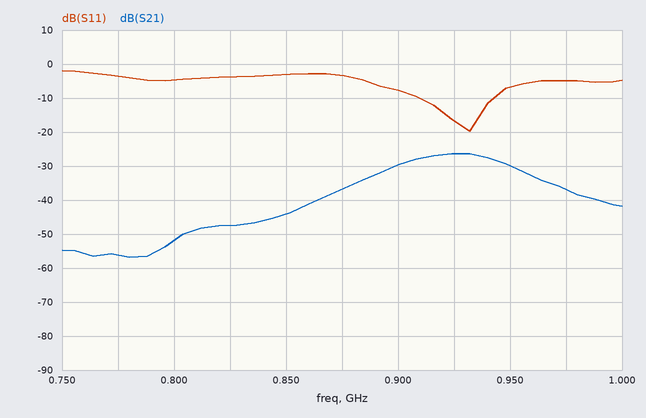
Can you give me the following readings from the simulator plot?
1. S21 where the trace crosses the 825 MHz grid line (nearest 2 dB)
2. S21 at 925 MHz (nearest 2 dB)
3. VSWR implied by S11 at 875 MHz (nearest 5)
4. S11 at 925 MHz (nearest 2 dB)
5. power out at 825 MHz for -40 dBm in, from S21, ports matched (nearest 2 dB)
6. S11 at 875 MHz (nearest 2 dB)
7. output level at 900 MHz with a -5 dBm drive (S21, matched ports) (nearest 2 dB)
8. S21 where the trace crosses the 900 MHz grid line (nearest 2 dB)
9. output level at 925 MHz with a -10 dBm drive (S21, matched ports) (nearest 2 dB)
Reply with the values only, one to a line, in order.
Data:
-48 dB
-26 dB
5
-16 dB
-88 dBm
-4 dB
-34 dBm
-30 dB
-36 dBm
